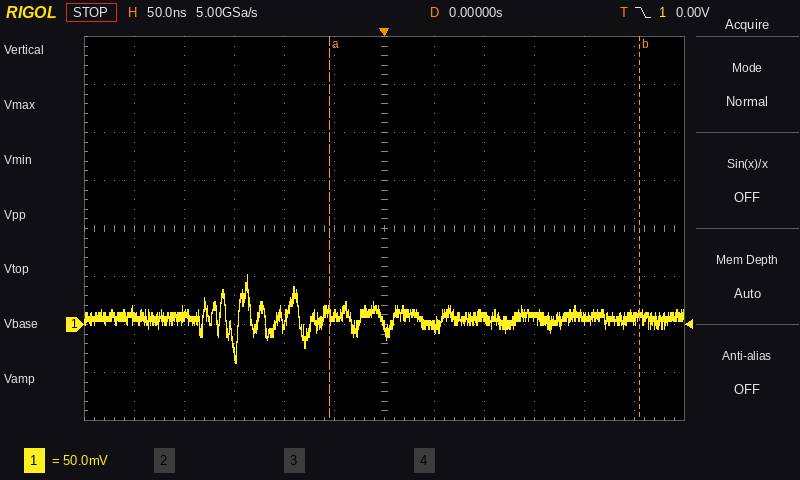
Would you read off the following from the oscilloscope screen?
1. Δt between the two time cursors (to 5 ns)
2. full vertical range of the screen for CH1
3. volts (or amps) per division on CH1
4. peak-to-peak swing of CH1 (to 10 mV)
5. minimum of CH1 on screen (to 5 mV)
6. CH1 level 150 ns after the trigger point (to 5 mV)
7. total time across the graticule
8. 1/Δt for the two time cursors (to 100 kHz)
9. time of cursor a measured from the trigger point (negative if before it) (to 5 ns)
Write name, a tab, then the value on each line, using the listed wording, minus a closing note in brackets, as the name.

Δt between the two time cursors	310 ns
full vertical range of the screen for CH1	400 mV
volts (or amps) per division on CH1	50 mV
peak-to-peak swing of CH1	90 mV
minimum of CH1 on screen	-40 mV
CH1 level 150 ns after the trigger point	10 mV
total time across the graticule	600 ns
1/Δt for the two time cursors	3.2 MHz
time of cursor a measured from the trigger point (negative if before it)	-55 ns
